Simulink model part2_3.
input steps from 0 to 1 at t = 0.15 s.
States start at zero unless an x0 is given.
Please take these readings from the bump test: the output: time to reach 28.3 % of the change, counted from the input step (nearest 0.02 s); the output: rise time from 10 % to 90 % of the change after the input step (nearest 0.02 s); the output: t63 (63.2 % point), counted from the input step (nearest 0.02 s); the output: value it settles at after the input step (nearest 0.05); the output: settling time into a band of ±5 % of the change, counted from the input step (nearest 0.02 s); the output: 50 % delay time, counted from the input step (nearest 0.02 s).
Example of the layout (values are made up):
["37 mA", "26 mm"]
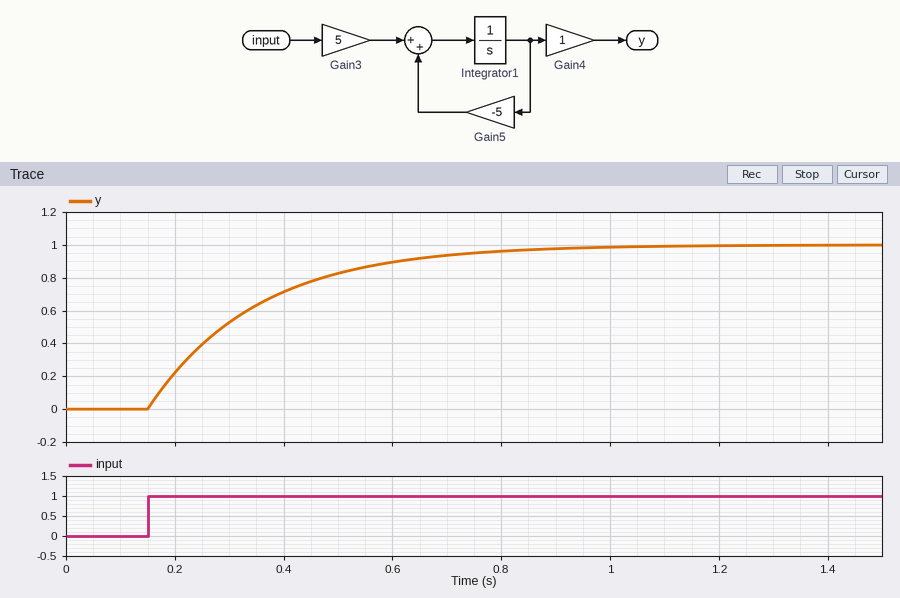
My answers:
["0.06 s", "0.44 s", "0.20 s", "1.00", "0.60 s", "0.14 s"]
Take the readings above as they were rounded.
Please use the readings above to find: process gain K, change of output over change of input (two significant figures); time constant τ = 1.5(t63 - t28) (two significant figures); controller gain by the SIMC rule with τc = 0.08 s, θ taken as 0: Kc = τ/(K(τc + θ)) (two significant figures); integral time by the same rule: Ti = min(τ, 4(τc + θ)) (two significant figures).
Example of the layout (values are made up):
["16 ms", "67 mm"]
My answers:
["1.0", "0.21 s", "2.6", "0.21 s"]
